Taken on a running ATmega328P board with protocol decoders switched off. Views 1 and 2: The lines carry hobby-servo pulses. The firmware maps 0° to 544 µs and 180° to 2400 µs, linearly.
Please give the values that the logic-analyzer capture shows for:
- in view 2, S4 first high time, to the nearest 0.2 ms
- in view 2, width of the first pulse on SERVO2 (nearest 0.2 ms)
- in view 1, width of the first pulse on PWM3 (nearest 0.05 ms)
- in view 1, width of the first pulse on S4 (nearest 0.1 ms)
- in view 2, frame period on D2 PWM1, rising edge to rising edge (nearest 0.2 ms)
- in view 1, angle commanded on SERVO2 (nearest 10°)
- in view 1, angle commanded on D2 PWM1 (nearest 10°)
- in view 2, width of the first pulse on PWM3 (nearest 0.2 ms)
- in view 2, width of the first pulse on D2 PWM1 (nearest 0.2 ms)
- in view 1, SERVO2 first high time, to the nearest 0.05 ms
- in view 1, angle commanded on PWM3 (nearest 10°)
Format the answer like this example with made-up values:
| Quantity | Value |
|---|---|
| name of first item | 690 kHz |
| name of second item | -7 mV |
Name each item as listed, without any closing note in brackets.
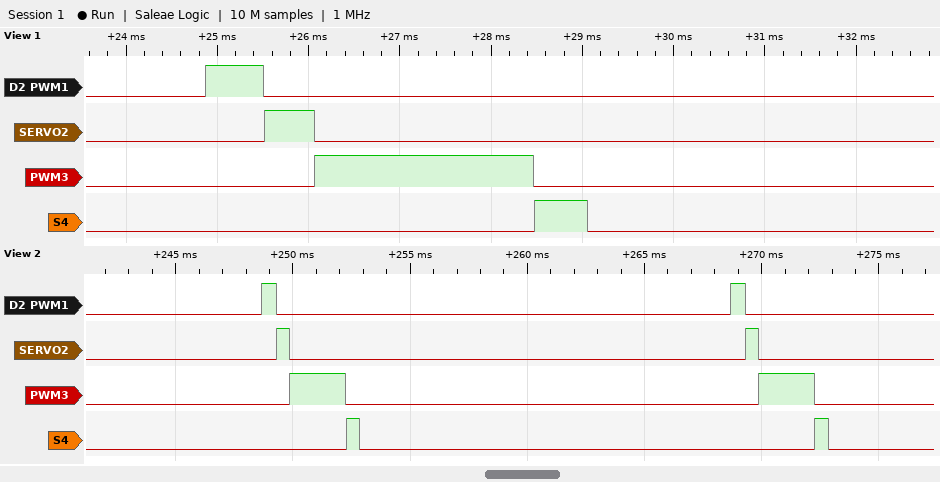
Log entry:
| Quantity | Value |
|---|---|
| in view 2, S4 first high time, to the nearest 0.2 ms | 0.6 ms |
| in view 2, width of the first pulse on SERVO2 | 0.6 ms |
| in view 1, width of the first pulse on PWM3 | 2.40 ms |
| in view 1, width of the first pulse on S4 | 0.6 ms |
| in view 2, frame period on D2 PWM1, rising edge to rising edge | 20.0 ms |
| in view 1, angle commanded on SERVO2 | 0° |
| in view 1, angle commanded on D2 PWM1 | 10° |
| in view 2, width of the first pulse on PWM3 | 2.4 ms |
| in view 2, width of the first pulse on D2 PWM1 | 0.6 ms |
| in view 1, SERVO2 first high time, to the nearest 0.05 ms | 0.55 ms |
| in view 1, angle commanded on PWM3 | 180° |
